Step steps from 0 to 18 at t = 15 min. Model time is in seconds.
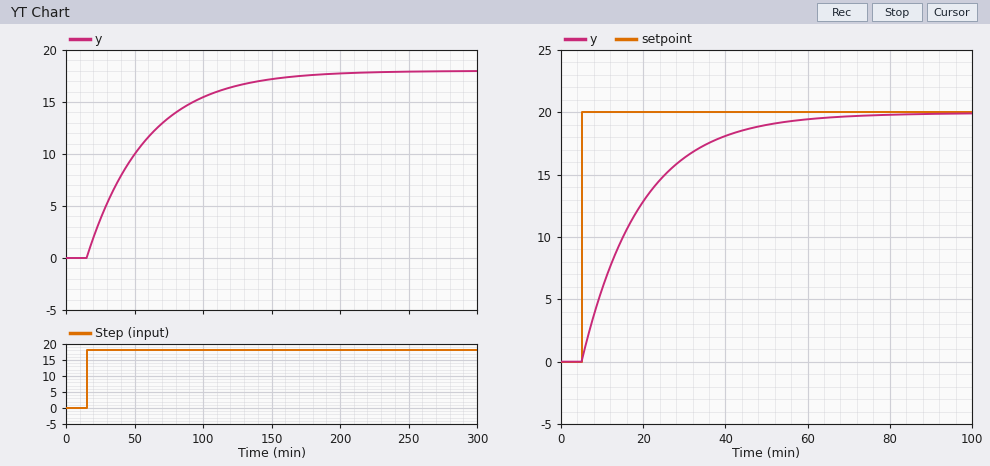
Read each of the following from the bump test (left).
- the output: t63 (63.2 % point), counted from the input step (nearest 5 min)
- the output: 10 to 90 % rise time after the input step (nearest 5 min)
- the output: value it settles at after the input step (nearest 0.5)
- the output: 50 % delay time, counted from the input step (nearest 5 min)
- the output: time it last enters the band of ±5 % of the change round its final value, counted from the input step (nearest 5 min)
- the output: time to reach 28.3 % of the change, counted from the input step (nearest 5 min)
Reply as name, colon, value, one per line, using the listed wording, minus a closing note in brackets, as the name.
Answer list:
the output: t63 (63.2 % point), counted from the input step: 45 min
the output: 10 to 90 % rise time after the input step: 95 min
the output: value it settles at after the input step: 18.0
the output: 50 % delay time, counted from the input step: 30 min
the output: time it last enters the band of ±5 % of the change round its final value, counted from the input step: 130 min
the output: time to reach 28.3 % of the change, counted from the input step: 15 min
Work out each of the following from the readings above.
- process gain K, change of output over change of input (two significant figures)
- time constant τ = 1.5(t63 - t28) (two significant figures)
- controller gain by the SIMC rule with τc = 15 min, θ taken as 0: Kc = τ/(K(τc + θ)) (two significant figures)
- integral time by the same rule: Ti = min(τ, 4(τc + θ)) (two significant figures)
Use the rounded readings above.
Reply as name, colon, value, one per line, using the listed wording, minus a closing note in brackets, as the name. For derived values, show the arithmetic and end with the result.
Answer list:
process gain K, change of output over change of input: (18 - 0) / 18 = 1.0
time constant τ = 1.5(t63 - t28): 1.5 × (45 - 15) = 45 min
controller gain by the SIMC rule with τc = 15 min, θ taken as 0: Kc = τ/(K(τc + θ)): 45 / (1 × (15 + 0)) = 3.0
integral time by the same rule: Ti = min(τ, 4(τc + θ)): min(45, 4 × (15 + 0)) = 45 min
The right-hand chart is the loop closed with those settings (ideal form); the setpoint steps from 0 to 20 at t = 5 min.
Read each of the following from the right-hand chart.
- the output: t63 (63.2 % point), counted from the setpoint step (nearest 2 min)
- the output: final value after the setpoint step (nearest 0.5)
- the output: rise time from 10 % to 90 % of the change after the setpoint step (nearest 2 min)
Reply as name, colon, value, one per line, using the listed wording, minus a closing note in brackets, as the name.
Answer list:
the output: t63 (63.2 % point), counted from the setpoint step: 14 min
the output: final value after the setpoint step: 20.0
the output: rise time from 10 % to 90 % of the change after the setpoint step: 32 min
